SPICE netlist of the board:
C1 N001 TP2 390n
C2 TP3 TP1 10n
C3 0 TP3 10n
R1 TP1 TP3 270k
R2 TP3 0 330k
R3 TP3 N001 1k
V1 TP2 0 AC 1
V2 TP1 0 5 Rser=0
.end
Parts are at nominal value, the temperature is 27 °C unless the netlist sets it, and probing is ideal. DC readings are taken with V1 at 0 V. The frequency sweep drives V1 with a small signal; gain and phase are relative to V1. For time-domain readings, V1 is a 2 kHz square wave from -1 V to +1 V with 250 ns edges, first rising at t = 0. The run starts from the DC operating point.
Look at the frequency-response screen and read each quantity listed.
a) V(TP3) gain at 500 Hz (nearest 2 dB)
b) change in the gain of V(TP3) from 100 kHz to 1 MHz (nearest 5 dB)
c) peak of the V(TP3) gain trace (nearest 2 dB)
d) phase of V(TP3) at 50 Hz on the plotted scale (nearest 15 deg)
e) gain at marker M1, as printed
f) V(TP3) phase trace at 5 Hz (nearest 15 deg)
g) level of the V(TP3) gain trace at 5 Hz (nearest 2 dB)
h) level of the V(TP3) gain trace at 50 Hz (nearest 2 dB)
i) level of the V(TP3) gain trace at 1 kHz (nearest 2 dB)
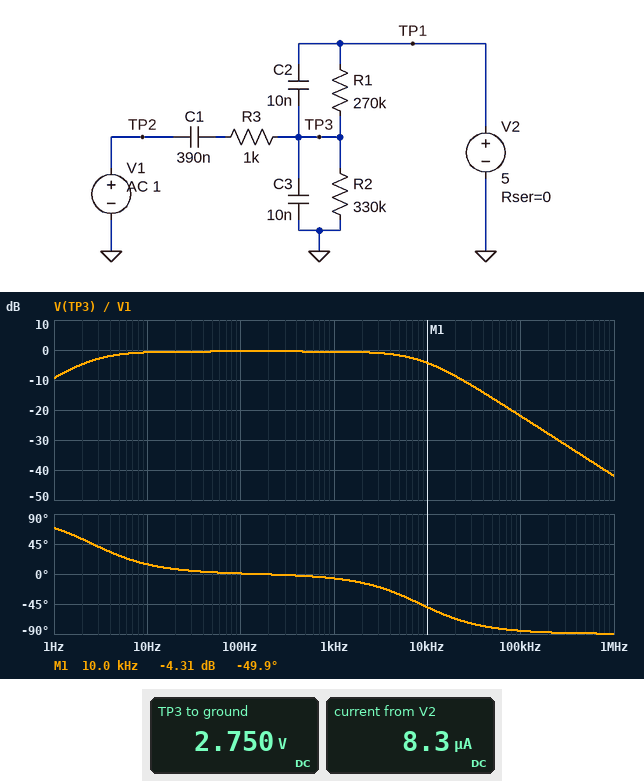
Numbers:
0 dB
-20 dB
0 dB
0 deg
-4.31 dB
30 deg
-2 dB
0 dB
0 dB
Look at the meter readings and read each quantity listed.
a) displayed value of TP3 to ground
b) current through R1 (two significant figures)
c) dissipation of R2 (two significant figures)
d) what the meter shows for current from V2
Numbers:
2.750 V
8.3 µA
23 µW
8.3 µA
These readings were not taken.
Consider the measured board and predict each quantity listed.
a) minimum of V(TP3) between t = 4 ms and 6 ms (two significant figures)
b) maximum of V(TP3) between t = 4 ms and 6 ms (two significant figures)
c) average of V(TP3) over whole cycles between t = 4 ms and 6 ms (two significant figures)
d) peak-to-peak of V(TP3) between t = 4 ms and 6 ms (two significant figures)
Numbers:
2.7 V
4.6 V
3.6 V
1.9 V
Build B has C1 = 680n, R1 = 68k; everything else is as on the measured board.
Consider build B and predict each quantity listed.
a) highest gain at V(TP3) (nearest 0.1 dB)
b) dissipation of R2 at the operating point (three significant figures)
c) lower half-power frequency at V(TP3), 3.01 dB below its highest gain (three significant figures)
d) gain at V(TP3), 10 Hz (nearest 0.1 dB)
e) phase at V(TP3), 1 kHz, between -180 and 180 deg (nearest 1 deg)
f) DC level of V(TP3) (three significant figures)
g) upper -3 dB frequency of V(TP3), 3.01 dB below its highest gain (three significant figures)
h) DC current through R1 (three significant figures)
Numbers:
-0.4 dB
52.1 µW
3.96 Hz
-1.0 dB
-7 deg
4.15 V
8.34 kHz
12.6 µA
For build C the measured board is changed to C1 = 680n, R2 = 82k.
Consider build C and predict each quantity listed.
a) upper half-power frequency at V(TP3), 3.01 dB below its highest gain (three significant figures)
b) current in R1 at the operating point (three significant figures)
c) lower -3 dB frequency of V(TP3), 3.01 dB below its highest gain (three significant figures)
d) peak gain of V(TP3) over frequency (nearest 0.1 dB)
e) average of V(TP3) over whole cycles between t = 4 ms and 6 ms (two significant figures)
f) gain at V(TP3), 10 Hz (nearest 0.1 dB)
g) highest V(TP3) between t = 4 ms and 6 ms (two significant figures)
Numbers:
8.32 kHz
14.2 µA
3.56 Hz
-0.4 dB
2.0 V
-0.9 dB
3.0 V
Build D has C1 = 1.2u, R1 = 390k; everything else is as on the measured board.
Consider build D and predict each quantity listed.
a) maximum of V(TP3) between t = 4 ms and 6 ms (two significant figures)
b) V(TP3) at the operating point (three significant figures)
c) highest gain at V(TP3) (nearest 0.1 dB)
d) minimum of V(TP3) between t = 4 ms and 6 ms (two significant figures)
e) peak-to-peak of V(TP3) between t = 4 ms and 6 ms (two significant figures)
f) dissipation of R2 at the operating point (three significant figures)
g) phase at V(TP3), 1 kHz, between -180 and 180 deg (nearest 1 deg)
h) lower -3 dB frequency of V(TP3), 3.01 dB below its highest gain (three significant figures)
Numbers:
4.2 V
2.29 V
-0.2 dB
2.3 V
2.0 V
15.9 µW
-7 deg
726 mHz
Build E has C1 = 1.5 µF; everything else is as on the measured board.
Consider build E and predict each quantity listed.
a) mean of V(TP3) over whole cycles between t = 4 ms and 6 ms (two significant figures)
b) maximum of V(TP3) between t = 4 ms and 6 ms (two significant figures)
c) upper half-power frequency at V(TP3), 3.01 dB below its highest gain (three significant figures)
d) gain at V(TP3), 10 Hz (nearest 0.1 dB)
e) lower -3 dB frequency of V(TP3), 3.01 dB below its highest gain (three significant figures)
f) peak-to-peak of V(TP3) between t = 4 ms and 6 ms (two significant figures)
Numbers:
3.7 V
4.7 V
8.12 kHz
-0.2 dB
700 mHz
2.0 V
